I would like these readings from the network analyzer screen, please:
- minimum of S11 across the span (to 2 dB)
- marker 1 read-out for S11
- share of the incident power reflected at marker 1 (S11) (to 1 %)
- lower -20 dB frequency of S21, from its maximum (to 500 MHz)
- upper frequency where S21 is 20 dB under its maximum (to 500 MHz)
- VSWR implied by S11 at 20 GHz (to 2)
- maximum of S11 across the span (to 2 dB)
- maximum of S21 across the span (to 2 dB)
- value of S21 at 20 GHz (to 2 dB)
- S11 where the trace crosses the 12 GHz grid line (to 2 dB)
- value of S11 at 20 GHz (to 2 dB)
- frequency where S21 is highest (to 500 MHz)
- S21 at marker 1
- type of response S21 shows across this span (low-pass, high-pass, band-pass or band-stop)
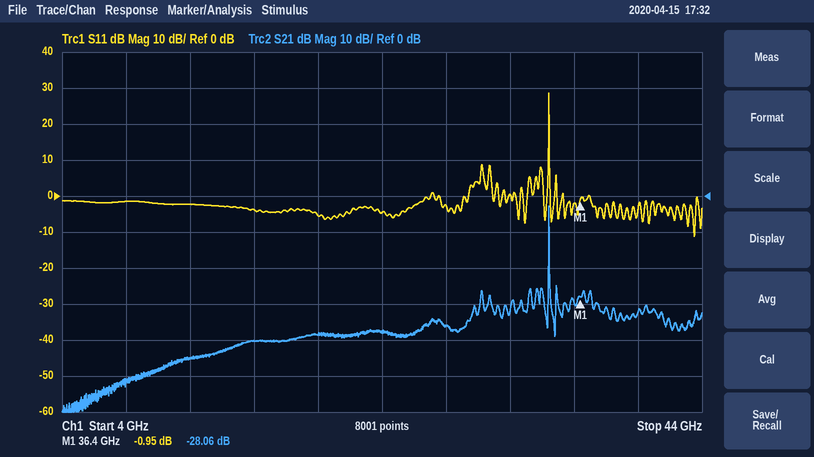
-12 dB
-0.95 dB
80 %
34.5 GHz
34.5 GHz
4
28 dB
-2 dB
-38 dB
-2 dB
-6 dB
34.5 GHz
-28.06 dB
band-pass
